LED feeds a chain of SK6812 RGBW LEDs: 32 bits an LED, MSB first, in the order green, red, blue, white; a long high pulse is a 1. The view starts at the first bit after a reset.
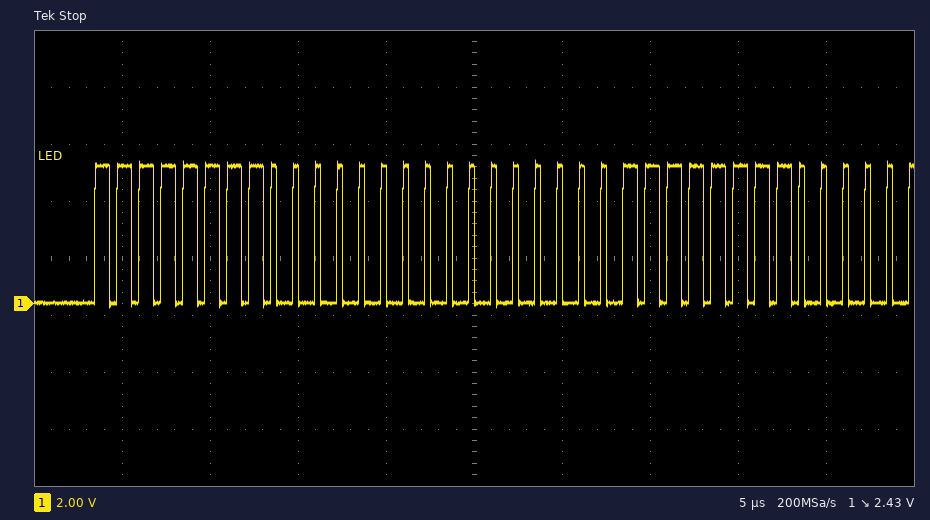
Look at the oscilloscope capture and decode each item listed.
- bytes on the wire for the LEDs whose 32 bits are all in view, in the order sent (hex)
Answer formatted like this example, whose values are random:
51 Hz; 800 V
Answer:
FF 00 00 FF
